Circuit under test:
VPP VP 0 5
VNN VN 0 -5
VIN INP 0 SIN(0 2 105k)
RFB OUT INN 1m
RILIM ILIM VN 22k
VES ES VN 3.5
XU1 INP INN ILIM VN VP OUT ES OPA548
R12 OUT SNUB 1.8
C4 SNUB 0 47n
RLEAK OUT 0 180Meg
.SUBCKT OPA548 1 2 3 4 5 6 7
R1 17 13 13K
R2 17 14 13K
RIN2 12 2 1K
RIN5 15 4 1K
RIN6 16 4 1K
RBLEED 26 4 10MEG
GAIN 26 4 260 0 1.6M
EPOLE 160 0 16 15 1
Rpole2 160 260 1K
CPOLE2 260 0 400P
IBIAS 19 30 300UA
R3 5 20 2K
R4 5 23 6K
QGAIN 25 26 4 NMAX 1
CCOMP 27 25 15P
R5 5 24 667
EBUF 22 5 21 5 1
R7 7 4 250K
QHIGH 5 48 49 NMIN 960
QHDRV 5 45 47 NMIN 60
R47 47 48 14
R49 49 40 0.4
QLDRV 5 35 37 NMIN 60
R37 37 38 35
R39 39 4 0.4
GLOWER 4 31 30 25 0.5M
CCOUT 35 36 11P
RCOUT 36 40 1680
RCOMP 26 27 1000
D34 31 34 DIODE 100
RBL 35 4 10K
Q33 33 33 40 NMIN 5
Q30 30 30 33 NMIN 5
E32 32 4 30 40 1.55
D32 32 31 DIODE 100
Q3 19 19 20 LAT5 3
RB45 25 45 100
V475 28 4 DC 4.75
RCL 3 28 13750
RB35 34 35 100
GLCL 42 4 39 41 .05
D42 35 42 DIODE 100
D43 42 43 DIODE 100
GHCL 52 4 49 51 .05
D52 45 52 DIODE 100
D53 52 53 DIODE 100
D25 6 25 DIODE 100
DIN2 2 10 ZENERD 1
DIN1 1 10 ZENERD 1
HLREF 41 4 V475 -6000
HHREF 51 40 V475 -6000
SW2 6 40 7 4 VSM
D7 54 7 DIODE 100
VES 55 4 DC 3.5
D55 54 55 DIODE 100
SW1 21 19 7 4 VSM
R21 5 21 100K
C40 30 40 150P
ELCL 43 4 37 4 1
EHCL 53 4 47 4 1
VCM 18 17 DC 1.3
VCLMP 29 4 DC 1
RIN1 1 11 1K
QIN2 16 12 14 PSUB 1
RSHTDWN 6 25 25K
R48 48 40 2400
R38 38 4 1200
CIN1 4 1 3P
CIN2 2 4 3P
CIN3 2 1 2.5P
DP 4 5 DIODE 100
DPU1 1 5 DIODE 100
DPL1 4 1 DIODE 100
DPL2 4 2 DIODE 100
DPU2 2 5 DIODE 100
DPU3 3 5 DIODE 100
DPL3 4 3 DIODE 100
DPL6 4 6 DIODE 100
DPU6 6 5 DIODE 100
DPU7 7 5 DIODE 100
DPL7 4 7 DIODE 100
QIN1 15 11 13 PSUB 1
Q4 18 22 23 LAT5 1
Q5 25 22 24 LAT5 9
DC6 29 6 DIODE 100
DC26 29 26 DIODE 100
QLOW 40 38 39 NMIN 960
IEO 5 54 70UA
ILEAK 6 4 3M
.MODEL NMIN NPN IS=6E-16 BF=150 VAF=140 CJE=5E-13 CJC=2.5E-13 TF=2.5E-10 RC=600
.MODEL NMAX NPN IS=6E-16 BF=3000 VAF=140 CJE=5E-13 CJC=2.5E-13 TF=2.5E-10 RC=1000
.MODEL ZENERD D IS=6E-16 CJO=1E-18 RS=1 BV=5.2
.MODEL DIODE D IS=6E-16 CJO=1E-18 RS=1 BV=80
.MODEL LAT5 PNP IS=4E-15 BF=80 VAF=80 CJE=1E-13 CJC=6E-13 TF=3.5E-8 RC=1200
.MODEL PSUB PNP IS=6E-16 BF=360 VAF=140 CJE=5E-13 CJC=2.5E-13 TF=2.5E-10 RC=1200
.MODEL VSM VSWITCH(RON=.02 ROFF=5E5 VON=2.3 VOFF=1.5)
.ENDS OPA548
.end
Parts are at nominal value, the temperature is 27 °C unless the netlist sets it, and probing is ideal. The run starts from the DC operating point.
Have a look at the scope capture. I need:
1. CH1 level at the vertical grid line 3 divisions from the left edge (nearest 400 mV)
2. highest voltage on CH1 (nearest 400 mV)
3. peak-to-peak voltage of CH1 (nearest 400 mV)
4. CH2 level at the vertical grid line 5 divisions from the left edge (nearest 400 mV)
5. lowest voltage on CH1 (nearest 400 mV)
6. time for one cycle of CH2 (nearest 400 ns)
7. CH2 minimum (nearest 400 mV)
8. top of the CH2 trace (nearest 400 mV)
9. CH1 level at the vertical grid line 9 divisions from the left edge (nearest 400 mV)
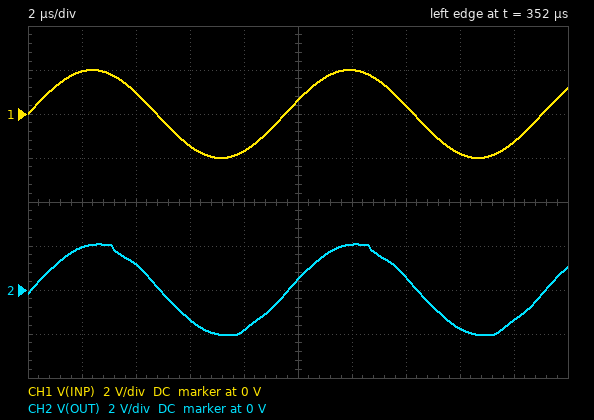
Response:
-1.6 V
2.0 V
4.0 V
400 mV
-2.0 V
9.6 µs
-2.0 V
2.0 V
-1.2 V
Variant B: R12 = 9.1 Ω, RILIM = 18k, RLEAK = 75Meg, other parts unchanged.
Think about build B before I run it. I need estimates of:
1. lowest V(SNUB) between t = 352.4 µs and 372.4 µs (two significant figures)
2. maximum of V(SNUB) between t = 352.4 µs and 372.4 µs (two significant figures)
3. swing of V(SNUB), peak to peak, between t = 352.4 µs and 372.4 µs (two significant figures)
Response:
-2.0 V
2.0 V
4.0 V
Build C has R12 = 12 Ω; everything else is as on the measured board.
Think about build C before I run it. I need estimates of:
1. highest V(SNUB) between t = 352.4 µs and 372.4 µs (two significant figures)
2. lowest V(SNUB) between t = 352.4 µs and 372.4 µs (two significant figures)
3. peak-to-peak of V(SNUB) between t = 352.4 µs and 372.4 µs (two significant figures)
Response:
1.9 V
-1.9 V
3.9 V
